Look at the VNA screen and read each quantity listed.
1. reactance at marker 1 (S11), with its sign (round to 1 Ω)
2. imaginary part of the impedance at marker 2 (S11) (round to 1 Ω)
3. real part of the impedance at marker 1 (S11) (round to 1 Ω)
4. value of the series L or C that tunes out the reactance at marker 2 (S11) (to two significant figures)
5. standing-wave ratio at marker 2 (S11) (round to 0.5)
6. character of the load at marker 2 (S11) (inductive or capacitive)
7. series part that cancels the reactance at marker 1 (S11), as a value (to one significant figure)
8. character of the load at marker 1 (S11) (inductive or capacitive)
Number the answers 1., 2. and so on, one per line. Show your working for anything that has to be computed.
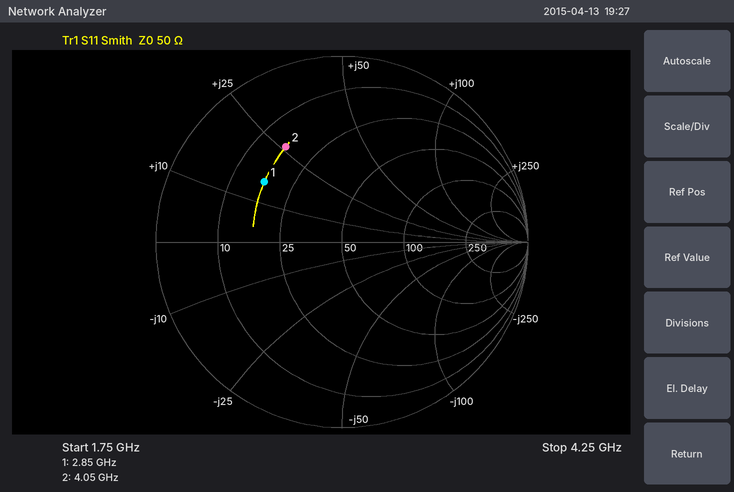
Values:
1. +15 Ω
2. +26 Ω
3. 17 Ω
4. C = 1/(2π × 4.05 GHz × 26 Ω) ≈ 1.5 pF
5. 4.0
6. inductive
7. C = 1/(2π × 2.85 GHz × 15 Ω) ≈ 4 pF
8. inductive
